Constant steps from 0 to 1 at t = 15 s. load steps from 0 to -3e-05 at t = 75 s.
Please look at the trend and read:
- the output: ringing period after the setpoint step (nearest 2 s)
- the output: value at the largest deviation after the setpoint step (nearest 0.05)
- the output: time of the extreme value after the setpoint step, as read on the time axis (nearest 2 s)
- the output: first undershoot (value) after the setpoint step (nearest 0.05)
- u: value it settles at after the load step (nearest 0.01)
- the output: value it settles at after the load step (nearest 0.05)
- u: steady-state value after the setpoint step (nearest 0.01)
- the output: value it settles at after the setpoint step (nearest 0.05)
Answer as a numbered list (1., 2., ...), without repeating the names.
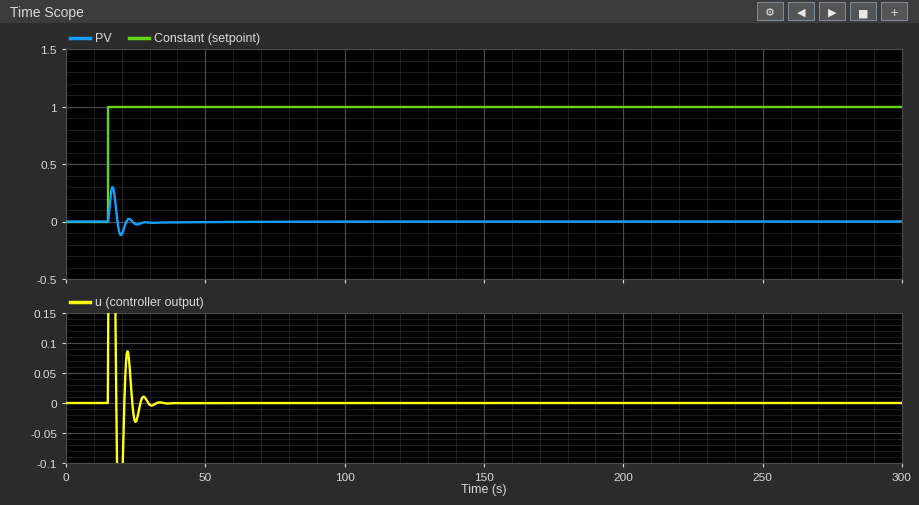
1. 6 s
2. 0.30
3. 16 s
4. -0.10
5. 0.00
6. 0.00
7. 0.00
8. 0.00
